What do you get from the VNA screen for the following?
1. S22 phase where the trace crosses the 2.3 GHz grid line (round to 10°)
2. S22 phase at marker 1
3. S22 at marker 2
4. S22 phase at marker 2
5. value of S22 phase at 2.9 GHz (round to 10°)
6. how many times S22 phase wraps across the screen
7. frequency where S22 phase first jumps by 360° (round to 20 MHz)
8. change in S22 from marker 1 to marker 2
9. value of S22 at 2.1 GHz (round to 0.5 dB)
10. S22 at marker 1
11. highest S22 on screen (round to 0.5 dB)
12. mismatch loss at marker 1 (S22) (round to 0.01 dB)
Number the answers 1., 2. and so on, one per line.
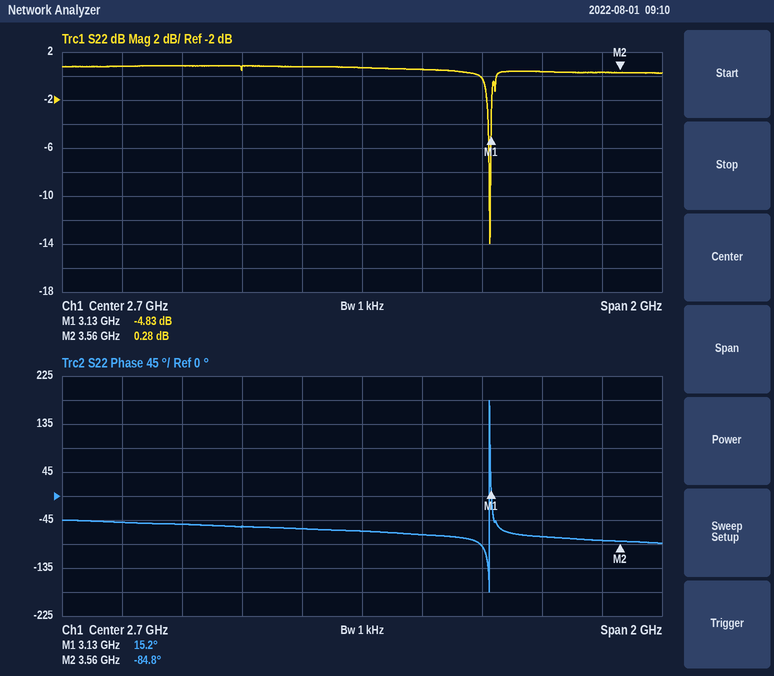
1. -60°
2. 15.2°
3. 0.28 dB
4. -84.8°
5. -70°
6. 1
7. 3.12 GHz
8. 5.11 dB
9. 1.0 dB
10. -4.83 dB
11. 1.0 dB
12. 1.73 dB
